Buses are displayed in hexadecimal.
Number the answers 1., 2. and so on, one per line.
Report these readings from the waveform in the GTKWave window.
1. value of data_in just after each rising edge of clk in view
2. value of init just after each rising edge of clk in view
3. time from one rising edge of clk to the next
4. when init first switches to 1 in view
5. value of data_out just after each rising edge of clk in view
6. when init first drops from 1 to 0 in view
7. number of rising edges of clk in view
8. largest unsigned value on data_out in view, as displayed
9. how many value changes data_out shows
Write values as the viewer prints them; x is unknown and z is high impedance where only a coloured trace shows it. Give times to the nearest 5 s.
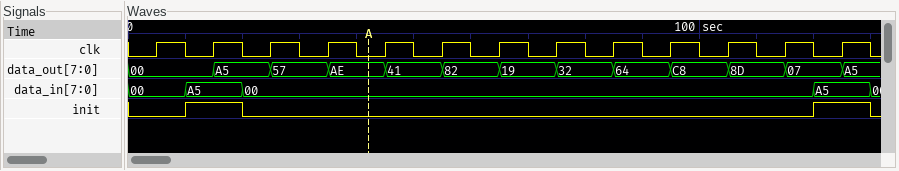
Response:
1. 00, A5, 00, 00, 00, 00, 00, 00, 00, 00, 00, 00, A5
2. 0 1 0 0 0 0 0 0 0 0 0 0 1
3. 10 s
4. 10 s
5. 00, A5, 57, AE, 41, 82, 19, 32, 64, C8, 8D, 07, A5
6. 20 s
7. 13
8. C8
9. 12
